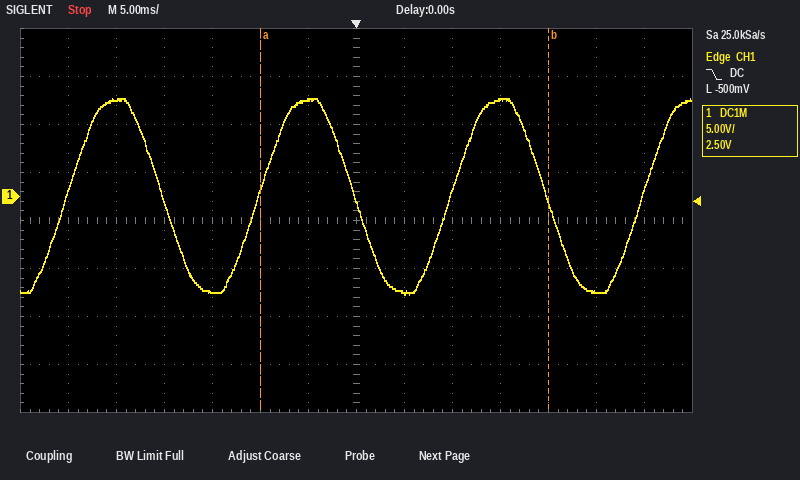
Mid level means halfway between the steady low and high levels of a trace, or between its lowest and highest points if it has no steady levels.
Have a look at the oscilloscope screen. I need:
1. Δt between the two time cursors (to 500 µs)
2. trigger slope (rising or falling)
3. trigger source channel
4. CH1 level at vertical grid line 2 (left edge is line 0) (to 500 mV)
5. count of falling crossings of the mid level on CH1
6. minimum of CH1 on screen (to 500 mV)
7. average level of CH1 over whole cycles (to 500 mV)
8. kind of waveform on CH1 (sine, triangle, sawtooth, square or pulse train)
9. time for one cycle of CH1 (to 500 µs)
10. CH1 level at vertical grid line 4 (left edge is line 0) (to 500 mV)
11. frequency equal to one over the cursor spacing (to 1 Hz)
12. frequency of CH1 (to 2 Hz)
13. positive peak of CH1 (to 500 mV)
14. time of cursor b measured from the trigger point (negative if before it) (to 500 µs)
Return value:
30.0 ms
falling
CH1
10.0 V
3
-10.0 V
0.0 V
sine
20.0 ms
-10.0 V
33 Hz
50 Hz
10.0 V
+20.0 ms
